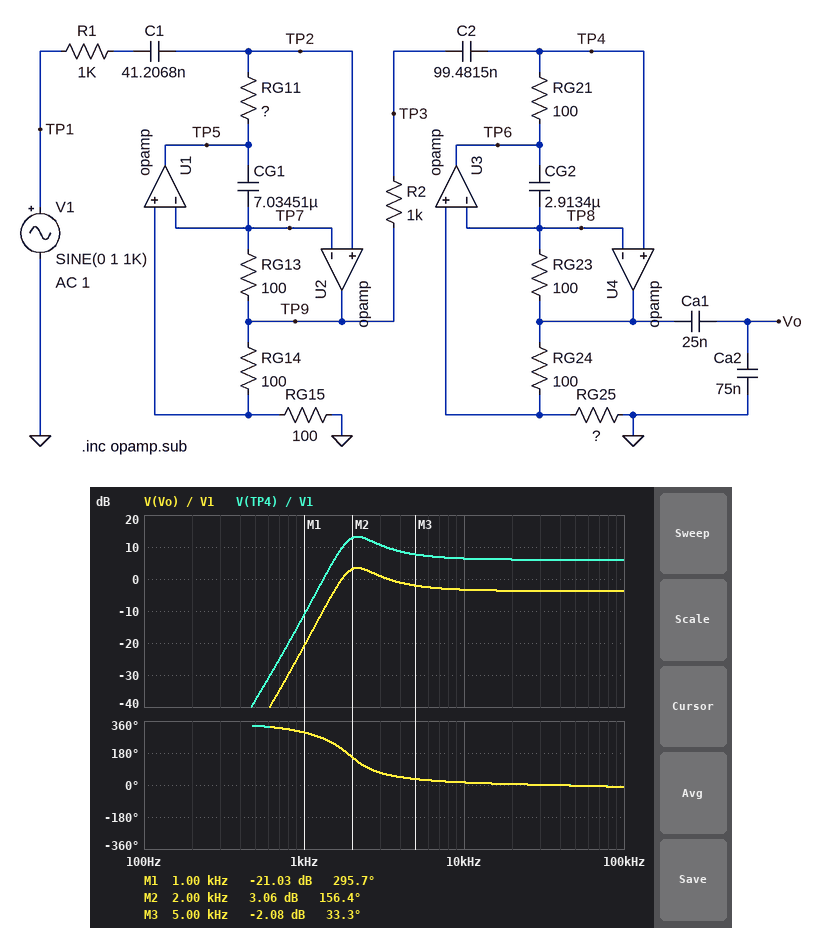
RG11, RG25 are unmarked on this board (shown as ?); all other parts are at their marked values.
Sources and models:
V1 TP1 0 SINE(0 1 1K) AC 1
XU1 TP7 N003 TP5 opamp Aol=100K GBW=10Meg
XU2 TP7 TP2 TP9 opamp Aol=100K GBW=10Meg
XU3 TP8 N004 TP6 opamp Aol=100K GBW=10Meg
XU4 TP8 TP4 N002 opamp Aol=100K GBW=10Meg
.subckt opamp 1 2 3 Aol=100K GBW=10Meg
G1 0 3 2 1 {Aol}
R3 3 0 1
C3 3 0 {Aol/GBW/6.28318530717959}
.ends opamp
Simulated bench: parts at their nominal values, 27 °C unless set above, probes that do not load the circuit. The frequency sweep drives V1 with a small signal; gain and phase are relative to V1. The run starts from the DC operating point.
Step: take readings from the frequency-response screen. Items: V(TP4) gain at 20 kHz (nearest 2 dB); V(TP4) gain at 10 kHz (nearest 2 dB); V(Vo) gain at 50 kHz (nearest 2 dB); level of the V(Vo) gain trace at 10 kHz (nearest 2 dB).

6 dB
6 dB
-4 dB
-4 dB
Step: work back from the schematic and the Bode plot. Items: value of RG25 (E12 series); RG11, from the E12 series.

330 Ω
220 Ω
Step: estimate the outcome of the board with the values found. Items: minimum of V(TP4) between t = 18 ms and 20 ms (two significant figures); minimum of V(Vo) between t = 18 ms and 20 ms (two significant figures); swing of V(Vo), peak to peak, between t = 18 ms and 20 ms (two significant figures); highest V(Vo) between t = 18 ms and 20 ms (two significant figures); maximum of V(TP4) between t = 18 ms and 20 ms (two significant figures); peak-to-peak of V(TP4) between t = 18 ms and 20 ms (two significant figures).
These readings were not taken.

-270 mV
-89 mV
180 mV
89 mV
270 mV
550 mV
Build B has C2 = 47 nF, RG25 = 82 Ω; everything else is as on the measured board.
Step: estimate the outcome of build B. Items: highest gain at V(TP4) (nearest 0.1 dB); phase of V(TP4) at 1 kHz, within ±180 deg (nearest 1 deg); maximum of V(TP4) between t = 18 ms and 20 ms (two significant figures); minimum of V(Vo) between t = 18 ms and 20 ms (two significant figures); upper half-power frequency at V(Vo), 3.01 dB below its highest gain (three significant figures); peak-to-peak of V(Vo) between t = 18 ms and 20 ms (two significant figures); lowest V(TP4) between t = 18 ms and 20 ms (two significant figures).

6.2 dB
-36 deg
28 mV
-16 mV
360 kHz
31 mV
-28 mV
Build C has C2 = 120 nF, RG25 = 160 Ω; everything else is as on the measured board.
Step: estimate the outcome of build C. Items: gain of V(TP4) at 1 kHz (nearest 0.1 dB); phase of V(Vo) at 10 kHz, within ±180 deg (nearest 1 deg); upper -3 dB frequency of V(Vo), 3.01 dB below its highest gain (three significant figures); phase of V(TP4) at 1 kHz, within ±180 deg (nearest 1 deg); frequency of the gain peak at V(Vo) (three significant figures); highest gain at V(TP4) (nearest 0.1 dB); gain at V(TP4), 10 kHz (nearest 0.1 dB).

-17.7 dB
24 deg
198 kHz
-63 deg
2.37 kHz
8.4 dB
6.2 dB
